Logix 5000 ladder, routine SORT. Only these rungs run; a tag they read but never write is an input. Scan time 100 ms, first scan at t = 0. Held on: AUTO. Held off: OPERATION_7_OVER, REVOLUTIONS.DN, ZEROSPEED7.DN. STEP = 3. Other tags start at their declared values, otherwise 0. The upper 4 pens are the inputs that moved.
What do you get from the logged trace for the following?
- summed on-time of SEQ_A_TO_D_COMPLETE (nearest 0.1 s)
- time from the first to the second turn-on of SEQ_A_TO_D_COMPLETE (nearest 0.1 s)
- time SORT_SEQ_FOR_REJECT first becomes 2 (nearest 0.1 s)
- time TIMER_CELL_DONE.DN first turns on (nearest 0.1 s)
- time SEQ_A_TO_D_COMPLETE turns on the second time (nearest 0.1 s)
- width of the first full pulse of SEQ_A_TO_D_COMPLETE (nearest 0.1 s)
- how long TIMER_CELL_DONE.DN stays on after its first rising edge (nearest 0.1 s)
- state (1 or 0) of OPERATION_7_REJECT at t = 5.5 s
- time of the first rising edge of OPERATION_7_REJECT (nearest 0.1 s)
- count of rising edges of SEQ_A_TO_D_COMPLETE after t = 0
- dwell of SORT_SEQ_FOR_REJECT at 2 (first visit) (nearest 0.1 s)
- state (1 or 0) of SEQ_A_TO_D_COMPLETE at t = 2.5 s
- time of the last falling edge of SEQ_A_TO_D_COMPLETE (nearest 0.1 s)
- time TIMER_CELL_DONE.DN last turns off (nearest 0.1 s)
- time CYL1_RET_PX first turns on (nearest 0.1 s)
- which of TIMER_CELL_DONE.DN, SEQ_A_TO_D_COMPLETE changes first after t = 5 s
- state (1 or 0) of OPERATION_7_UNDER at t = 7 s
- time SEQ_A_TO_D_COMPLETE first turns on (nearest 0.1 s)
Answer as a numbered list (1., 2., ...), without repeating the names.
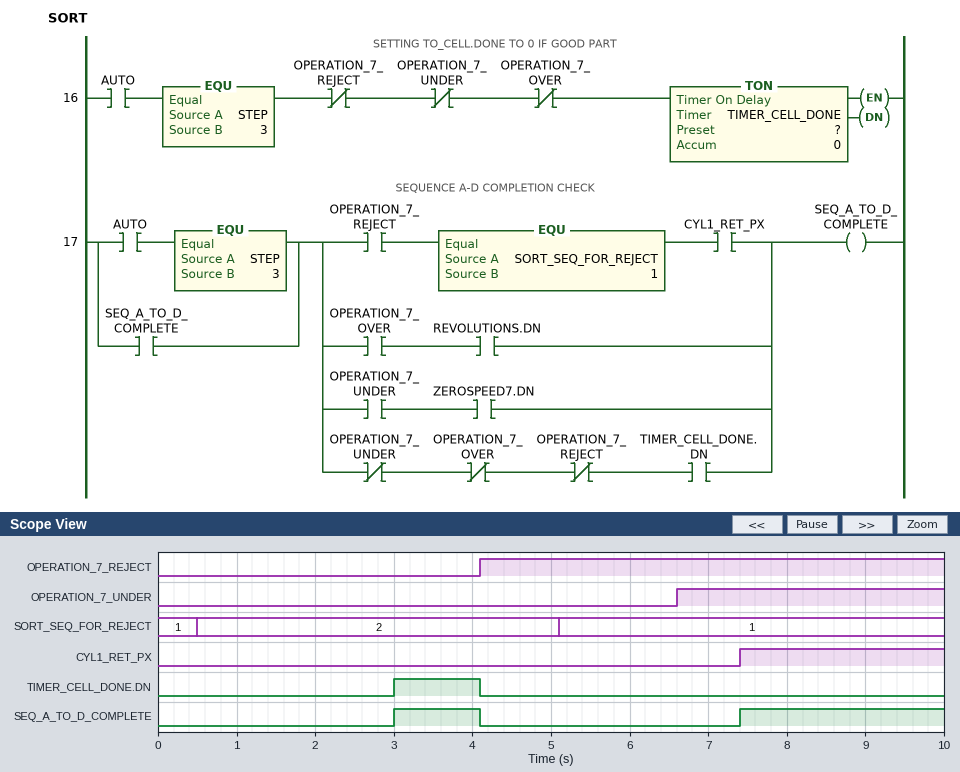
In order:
1. 3.7 s
2. 4.4 s
3. 0.5 s
4. 3.0 s
5. 7.4 s
6. 1.1 s
7. 1.1 s
8. 1
9. 4.1 s
10. 2
11. 4.6 s
12. 0
13. 4.1 s
14. 4.1 s
15. 7.4 s
16. SEQ_A_TO_D_COMPLETE
17. 1
18. 3.0 s
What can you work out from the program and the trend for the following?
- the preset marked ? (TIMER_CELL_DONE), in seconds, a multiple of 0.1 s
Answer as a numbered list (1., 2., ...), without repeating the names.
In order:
1. 3.0 s
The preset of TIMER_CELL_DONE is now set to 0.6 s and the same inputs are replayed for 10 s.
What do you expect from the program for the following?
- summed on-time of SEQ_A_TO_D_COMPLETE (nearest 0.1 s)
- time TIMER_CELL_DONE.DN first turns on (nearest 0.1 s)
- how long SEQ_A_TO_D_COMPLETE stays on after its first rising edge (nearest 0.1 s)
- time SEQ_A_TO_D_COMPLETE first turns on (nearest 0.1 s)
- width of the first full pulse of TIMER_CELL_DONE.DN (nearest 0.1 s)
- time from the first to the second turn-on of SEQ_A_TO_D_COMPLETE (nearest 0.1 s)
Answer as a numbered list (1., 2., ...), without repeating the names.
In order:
1. 6.1 s
2. 0.6 s
3. 3.5 s
4. 0.6 s
5. 3.5 s
6. 6.8 s
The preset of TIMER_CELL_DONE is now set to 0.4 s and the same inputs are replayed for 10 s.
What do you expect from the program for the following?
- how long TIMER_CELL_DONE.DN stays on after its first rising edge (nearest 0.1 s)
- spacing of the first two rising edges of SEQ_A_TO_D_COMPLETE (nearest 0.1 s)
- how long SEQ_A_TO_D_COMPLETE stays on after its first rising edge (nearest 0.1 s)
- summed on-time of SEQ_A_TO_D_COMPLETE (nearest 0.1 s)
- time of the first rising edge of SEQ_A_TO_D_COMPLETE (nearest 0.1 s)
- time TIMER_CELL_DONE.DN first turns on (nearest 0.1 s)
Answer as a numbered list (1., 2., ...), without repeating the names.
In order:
1. 3.7 s
2. 7.0 s
3. 3.7 s
4. 6.3 s
5. 0.4 s
6. 0.4 s
